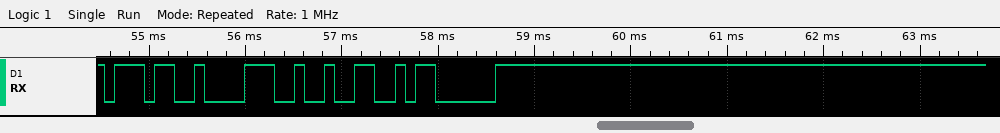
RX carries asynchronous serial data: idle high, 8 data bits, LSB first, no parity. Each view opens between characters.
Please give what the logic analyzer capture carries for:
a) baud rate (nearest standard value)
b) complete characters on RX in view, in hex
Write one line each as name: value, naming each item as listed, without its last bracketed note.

baud rate: 9600 baud
complete characters on RX in view, in hex: 37, 38, 32, 03
